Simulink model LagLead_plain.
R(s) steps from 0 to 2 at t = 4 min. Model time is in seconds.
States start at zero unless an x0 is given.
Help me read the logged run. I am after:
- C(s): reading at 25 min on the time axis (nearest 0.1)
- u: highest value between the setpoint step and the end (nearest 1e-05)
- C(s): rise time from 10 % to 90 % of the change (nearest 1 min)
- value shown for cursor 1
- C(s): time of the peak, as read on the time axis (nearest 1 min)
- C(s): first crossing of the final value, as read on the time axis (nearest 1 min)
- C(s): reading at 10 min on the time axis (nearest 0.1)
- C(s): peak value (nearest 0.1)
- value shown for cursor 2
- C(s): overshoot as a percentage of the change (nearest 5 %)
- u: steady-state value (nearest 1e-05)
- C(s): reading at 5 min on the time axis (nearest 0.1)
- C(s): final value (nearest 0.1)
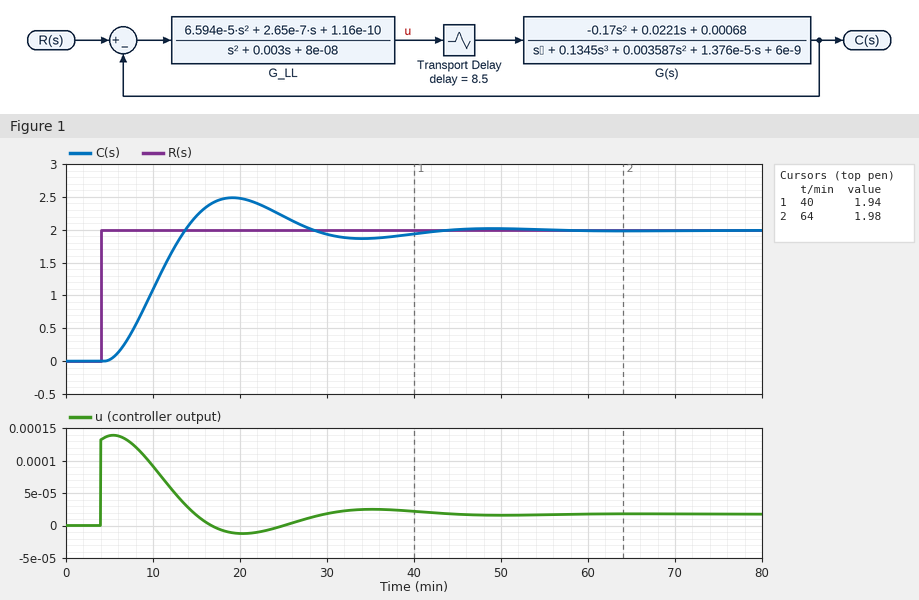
2.2
0.00014
6 min
1.94
19 min
14 min
1.1
2.5
1.98
25 %
0.00002
0.0
2.0
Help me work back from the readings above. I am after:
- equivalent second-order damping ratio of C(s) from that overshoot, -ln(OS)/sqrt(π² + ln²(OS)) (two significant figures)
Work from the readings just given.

0.40
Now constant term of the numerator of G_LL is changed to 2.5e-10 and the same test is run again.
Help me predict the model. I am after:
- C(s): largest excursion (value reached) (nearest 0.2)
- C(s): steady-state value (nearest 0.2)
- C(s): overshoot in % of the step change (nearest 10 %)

2.8
2.0
40 %
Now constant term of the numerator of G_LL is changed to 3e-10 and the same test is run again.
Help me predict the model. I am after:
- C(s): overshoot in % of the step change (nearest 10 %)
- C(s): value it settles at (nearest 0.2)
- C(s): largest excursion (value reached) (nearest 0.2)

40 %
2.0
2.8
